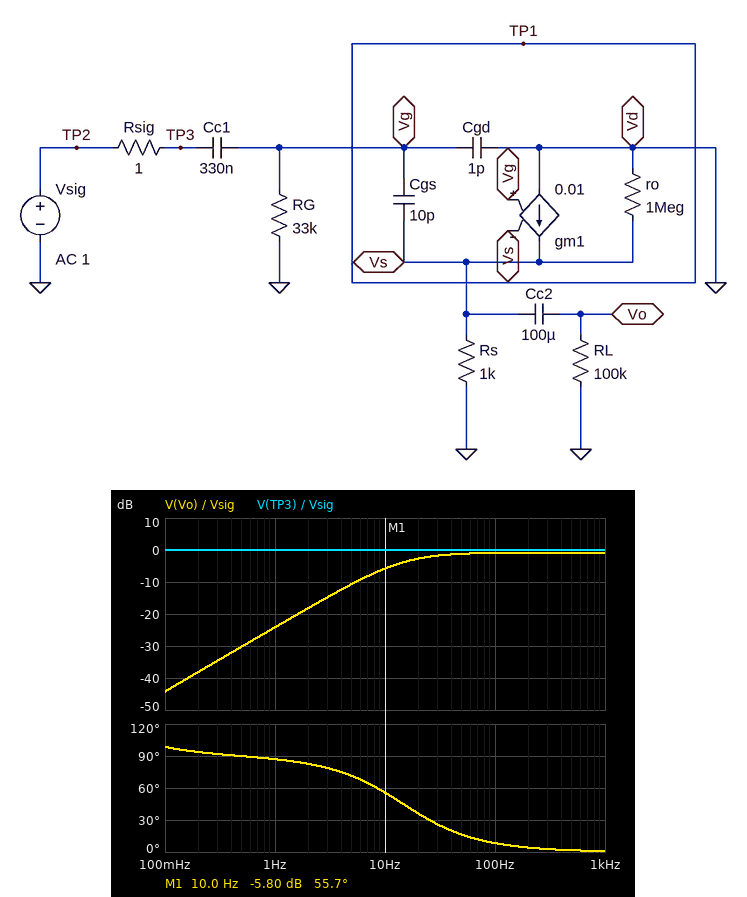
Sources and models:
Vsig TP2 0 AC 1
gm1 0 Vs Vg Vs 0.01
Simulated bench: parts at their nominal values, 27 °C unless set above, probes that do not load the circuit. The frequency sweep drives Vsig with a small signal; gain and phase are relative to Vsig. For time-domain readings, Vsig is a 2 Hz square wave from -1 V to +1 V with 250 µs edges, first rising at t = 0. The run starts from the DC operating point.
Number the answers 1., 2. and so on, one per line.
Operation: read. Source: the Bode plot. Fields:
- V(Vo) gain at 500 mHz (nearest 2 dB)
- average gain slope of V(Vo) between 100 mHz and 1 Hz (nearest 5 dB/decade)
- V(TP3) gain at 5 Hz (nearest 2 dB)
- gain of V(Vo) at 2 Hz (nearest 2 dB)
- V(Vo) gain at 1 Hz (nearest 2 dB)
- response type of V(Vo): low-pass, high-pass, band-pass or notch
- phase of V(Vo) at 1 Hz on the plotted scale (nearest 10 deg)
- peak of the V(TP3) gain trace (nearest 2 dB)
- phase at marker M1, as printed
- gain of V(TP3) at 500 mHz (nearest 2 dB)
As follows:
1. -30 dB
2. 20 dB/decade
3. 0 dB
4. -18 dB
5. -24 dB
6. high-pass
7. 90 deg
8. 0 dB
9. 55.7 deg
10. 0 dB
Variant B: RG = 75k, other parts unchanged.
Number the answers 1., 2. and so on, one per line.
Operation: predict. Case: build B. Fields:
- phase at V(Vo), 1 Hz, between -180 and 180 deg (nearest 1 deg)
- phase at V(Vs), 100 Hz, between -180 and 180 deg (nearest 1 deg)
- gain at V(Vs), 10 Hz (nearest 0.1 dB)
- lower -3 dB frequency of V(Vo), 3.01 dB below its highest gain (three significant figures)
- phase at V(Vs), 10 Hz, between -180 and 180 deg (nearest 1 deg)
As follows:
1. 82 deg
2. 4 deg
3. -2.3 dB
4. 6.43 Hz
5. 33 deg
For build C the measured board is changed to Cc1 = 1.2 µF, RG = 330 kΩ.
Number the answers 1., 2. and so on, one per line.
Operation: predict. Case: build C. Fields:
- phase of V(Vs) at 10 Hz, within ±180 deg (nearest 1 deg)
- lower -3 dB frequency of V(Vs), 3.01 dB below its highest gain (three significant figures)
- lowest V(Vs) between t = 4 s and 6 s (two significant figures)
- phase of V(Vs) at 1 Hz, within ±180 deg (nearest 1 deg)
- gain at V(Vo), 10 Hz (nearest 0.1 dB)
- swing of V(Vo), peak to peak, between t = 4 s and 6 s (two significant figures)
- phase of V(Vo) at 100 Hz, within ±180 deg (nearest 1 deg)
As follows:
1. 2 deg
2. 402 mHz
3. -1.2 V
4. 22 deg
5. -0.8 dB
6. 2.4 V
7. 0 deg
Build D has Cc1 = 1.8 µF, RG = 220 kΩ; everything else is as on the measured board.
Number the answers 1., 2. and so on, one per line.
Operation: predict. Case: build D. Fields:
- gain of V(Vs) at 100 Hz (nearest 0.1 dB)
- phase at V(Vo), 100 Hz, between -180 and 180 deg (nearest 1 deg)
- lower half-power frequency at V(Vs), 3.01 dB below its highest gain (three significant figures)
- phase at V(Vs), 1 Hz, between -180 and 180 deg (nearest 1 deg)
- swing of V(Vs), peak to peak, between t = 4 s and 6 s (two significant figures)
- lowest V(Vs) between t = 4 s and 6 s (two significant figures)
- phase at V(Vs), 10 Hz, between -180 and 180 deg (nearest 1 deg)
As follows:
1. -0.8 dB
2. 0 deg
3. 402 mHz
4. 22 deg
5. 2.4 V
6. -1.2 V
7. 2 deg
